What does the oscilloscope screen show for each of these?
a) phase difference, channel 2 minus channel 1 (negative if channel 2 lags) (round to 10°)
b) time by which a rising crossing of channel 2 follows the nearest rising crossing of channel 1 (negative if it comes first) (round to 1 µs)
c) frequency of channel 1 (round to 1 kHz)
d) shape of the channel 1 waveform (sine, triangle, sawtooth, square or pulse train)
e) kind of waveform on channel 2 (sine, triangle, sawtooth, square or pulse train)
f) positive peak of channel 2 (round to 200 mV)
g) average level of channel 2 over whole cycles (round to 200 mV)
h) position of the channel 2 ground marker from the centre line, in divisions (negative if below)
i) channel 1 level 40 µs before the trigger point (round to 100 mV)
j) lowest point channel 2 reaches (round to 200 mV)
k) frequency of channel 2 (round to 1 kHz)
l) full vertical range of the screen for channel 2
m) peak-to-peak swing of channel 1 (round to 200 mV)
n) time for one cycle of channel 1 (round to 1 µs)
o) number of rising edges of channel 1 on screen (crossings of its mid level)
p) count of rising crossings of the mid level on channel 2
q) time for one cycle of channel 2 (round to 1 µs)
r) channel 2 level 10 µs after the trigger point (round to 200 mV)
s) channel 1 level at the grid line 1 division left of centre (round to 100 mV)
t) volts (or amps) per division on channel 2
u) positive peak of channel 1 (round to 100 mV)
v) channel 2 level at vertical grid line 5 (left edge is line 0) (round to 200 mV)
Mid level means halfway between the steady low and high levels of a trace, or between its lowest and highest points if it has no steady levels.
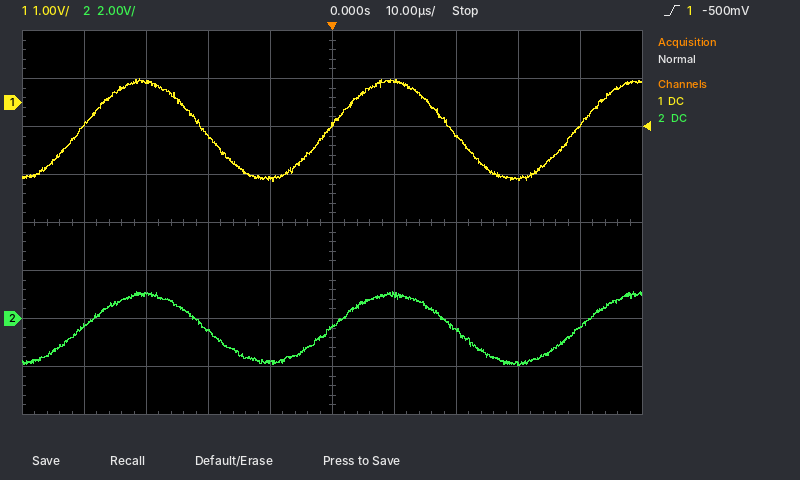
0°
0 µs
25 kHz
sine
sine
1.2 V
-400 mV
-2.0 div
-500 mV
-2.0 V
25 kHz
16 V
2.2 V
40 µs
3
3
40 µs
1.0 V
-1.6 V
2 V
500 mV
-400 mV
